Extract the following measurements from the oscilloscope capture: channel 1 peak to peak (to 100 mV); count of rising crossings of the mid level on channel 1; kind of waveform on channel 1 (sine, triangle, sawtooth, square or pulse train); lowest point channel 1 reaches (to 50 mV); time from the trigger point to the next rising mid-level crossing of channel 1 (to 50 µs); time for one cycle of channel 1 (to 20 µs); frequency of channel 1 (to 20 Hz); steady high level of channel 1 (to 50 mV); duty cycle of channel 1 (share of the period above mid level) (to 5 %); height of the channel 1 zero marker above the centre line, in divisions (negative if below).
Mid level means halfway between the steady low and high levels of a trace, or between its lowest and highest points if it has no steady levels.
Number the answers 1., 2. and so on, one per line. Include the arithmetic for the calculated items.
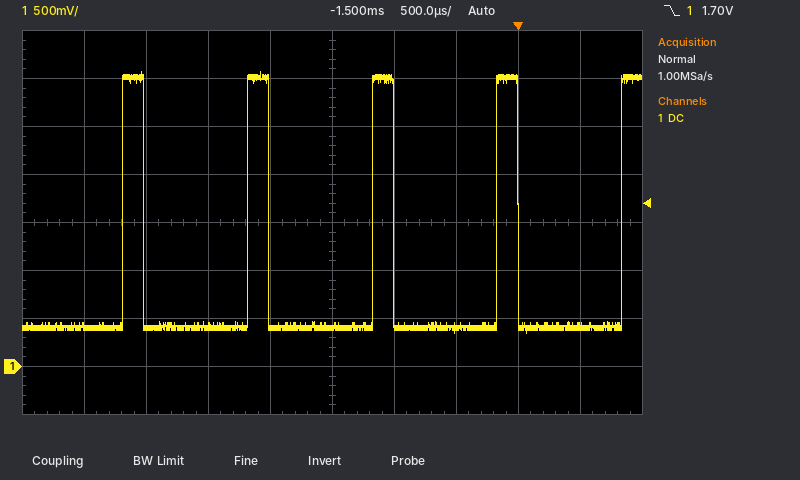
1. 2.70 V
2. 5
3. pulse train
4. 350 mV
5. 850 µs
6. 1.00 ms
7. 1 / 1.00 ms ≈ 1.00 kHz
8. 3.00 V
9. 15 %
10. -3.0 div
